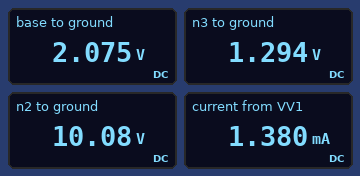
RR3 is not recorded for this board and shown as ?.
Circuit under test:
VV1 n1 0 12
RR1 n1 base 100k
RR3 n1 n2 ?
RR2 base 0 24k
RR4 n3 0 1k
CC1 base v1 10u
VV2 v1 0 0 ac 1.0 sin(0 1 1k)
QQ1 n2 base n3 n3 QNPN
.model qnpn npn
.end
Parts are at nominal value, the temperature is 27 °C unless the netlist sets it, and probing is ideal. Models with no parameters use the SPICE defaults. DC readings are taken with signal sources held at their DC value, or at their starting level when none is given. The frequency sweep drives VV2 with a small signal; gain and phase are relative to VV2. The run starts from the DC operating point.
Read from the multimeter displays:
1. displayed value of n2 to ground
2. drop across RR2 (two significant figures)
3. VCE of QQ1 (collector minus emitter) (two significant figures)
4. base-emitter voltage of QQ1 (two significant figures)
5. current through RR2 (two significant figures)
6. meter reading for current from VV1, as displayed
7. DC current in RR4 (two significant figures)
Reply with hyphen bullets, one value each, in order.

- 10.08 V
- 2.1 V
- 8.8 V
- 780 mV
- 86 µA
- 1.380 mA
- 1.3 mA
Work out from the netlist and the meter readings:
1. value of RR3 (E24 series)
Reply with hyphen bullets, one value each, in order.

- 1.5 kΩ
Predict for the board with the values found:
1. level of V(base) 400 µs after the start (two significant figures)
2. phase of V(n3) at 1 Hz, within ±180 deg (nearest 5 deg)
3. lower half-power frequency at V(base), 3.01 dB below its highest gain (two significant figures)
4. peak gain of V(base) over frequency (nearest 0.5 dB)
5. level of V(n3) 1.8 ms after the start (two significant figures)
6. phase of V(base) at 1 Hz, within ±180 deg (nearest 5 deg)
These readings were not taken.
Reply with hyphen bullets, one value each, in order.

- 2.7 V
- 45 deg
- 980 mHz
- 0 dB
- 370 mV
- 45 deg
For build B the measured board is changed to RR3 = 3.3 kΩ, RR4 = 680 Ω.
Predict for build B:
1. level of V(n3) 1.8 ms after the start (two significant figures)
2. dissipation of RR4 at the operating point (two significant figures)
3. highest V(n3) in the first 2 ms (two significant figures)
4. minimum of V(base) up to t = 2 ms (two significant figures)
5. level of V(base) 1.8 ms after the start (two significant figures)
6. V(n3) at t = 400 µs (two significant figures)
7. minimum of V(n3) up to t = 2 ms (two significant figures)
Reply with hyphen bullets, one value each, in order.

- 280 mV
- 2.1 mW
- 2.2 V
- 980 mV
- 1.0 V
- 1.8 V
- 230 mV
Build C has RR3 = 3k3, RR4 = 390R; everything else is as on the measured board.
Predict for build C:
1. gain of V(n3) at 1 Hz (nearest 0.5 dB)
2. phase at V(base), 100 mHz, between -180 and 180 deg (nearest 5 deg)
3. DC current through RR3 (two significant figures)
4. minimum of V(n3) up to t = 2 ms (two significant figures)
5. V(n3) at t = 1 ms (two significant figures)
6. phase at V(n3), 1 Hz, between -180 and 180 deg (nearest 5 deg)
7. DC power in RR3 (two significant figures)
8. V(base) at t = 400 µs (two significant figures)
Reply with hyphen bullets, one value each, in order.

- -4.0 dB
- 85 deg
- 2.6 mA
- 22 mV
- 970 mV
- 50 deg
- 22 mW
- 2.4 V
